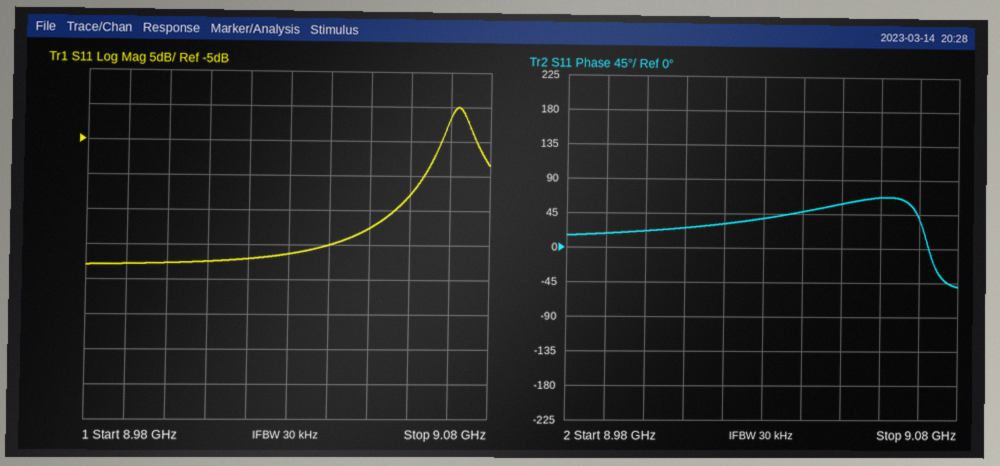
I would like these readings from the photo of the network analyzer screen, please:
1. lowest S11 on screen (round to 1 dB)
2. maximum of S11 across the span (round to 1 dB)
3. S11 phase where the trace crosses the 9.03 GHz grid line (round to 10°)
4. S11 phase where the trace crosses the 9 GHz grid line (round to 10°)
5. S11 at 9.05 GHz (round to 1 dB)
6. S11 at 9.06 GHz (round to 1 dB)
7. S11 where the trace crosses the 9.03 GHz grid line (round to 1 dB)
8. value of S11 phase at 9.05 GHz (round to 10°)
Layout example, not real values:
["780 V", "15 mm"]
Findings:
["-23 dB", "0 dB", "40°", "20°", "-18 dB", "-13 dB", "-21 dB", "60°"]
